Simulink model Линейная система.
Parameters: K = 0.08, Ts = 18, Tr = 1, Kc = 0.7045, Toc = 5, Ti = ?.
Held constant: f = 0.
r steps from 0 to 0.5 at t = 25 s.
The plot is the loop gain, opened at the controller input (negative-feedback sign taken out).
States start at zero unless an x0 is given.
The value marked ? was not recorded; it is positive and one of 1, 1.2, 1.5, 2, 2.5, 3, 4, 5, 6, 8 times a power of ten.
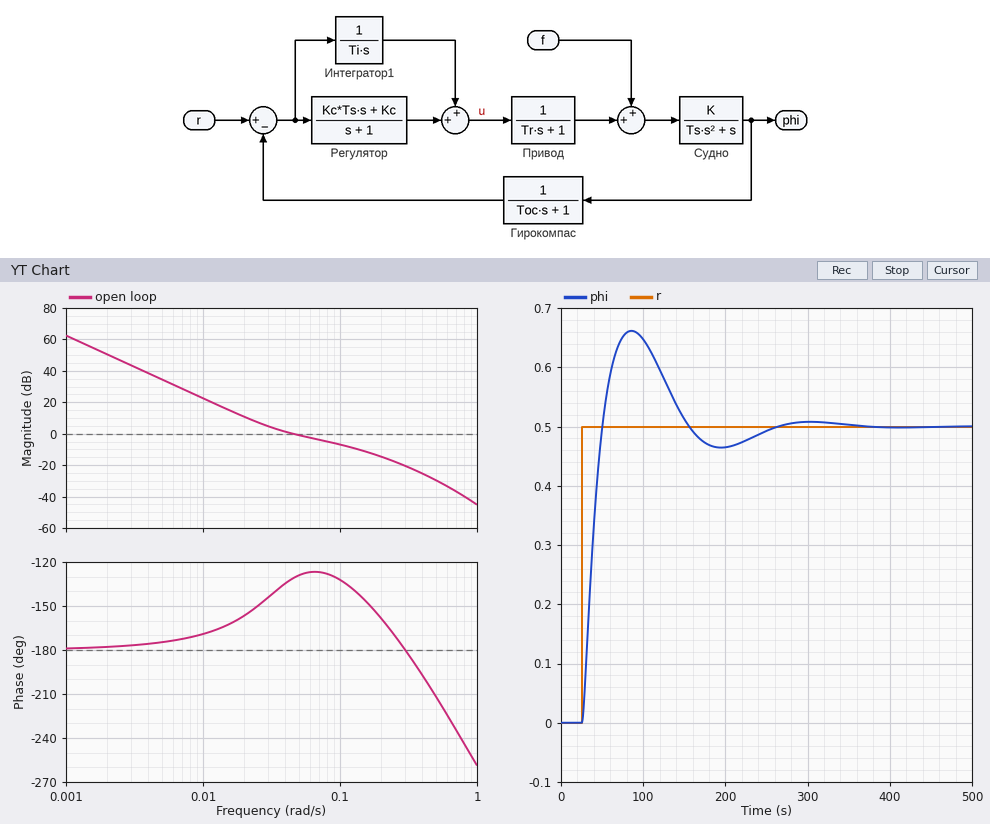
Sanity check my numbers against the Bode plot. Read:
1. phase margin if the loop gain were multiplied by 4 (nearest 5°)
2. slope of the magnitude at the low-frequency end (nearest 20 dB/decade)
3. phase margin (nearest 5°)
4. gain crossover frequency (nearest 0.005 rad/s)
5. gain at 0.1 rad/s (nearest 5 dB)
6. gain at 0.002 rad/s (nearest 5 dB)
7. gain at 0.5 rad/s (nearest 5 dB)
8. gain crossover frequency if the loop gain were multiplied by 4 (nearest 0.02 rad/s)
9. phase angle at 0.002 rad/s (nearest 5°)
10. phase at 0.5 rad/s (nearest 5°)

30°
-40 dB/decade
50°
0.045 rad/s
-5 dB
50 dB
-30 dB
0.16 rad/s
-180°
-210°
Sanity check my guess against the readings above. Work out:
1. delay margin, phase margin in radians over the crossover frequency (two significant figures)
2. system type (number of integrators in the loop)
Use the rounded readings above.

19 s
2
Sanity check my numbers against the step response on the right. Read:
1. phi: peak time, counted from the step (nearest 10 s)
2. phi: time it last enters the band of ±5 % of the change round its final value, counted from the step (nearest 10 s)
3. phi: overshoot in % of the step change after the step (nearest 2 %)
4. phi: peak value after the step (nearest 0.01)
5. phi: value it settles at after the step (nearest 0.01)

60 s
200 s
32 %
0.66
0.50
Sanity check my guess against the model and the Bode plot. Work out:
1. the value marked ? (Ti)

60
